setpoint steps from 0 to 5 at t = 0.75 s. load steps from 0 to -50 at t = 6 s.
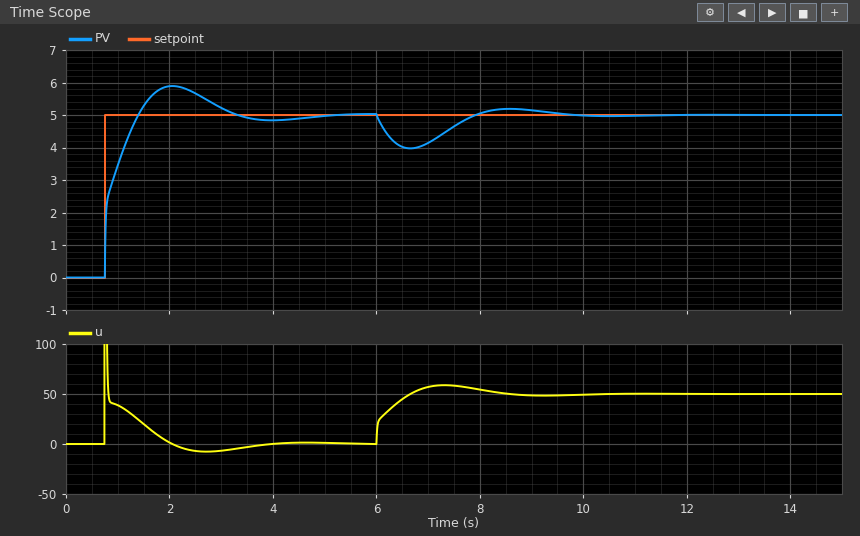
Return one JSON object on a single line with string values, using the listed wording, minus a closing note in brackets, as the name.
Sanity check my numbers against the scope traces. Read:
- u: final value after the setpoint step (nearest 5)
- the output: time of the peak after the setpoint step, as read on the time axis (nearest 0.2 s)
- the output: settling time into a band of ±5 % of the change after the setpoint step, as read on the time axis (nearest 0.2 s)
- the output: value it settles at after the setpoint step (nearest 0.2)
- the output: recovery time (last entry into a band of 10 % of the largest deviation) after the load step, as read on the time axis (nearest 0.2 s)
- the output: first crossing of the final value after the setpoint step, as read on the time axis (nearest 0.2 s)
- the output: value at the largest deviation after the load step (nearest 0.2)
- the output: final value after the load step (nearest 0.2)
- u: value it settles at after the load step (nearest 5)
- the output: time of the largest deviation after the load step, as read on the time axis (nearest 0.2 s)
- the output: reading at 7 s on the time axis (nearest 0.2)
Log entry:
{"u: final value after the setpoint step": "0", "the output: time of the peak after the setpoint step, as read on the time axis": "2.0 s", "the output: settling time into a band of ±5 % of the change after the setpoint step, as read on the time axis": "3.0 s", "the output: value it settles at after the setpoint step": "5.0", "the output: recovery time (last entry into a band of 10 % of the largest deviation) after the load step, as read on the time axis": "9.2 s", "the output: first crossing of the final value after the setpoint step, as read on the time axis": "1.4 s", "the output: value at the largest deviation after the load step": "4.0", "the output: final value after the load step": "5.0", "u: value it settles at after the load step": "50", "the output: time of the largest deviation after the load step, as read on the time axis": "6.6 s", "the output: reading at 7 s on the time axis": "4.2"}
